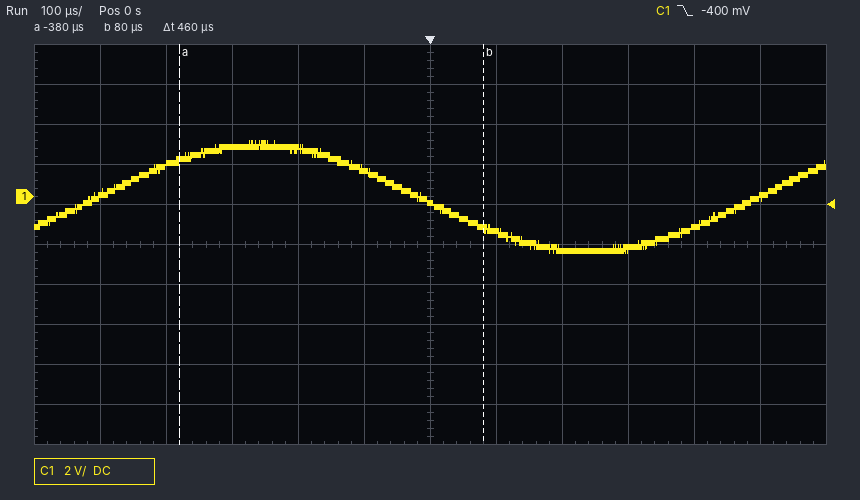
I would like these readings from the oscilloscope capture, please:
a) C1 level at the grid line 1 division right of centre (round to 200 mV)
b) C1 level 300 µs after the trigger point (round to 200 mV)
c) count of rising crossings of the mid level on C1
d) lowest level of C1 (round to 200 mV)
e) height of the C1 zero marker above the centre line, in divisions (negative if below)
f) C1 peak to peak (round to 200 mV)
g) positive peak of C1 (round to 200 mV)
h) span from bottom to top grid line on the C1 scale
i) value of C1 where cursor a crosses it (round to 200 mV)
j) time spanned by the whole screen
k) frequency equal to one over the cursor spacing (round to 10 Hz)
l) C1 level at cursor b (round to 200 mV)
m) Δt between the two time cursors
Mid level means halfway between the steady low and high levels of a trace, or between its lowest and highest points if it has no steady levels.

-1.8 V
-2.6 V
2
-2.8 V
+1.2 div
5.6 V
2.8 V
20 V
1.8 V
1.2 ms
2.17 kHz
-1.6 V
460 µs
